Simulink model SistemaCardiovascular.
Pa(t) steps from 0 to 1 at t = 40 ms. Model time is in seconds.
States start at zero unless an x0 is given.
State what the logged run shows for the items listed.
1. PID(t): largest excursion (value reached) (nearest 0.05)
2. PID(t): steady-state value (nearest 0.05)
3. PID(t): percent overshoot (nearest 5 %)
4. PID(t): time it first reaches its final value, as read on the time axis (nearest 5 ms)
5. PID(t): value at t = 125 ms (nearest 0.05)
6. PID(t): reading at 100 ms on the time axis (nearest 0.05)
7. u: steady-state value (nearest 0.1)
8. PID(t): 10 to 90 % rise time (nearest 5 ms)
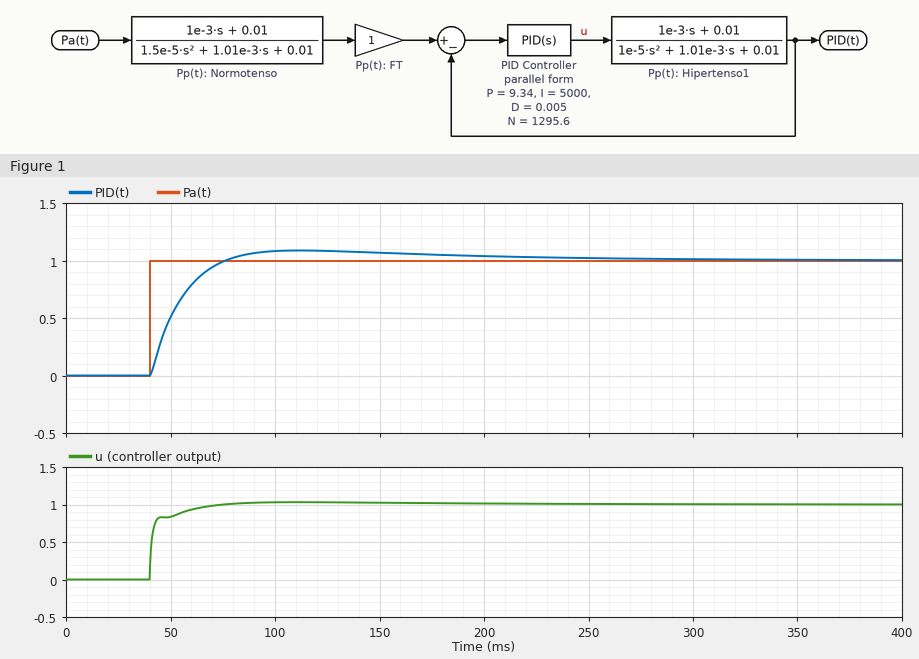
1.10
1.00
10 %
75 ms
1.10
1.10
1.0
25 ms
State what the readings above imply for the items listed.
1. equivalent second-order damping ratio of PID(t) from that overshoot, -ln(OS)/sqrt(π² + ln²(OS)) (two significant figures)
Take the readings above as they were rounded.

0.59
